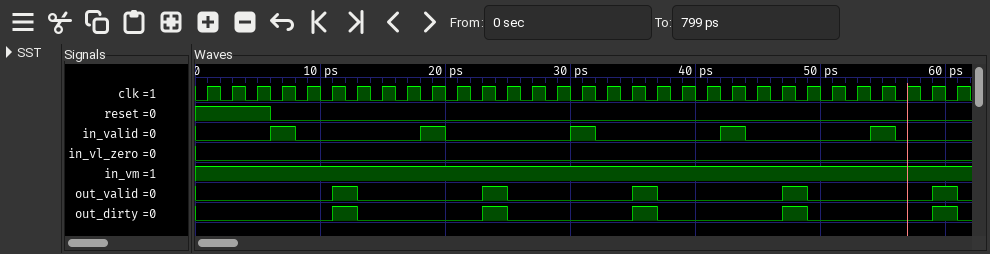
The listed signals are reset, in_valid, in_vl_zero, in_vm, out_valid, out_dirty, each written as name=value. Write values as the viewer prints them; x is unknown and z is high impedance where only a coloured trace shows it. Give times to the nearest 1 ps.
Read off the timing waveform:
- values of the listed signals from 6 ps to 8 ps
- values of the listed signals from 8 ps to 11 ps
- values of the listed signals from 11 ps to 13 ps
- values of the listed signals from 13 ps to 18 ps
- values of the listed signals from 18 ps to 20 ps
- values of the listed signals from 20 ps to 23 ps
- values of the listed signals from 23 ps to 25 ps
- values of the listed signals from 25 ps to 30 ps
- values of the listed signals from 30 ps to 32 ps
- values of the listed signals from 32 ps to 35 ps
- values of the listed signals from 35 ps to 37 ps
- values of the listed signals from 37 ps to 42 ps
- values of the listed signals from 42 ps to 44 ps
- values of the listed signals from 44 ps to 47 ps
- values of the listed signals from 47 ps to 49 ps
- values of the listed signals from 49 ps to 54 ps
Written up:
reset=0, in_valid=1, in_vl_zero=0, in_vm=1, out_valid=0, out_dirty=0
reset=0, in_valid=0, in_vl_zero=0, in_vm=1, out_valid=0, out_dirty=0
reset=0, in_valid=0, in_vl_zero=0, in_vm=1, out_valid=1, out_dirty=1
reset=0, in_valid=0, in_vl_zero=0, in_vm=1, out_valid=0, out_dirty=0
reset=0, in_valid=1, in_vl_zero=0, in_vm=1, out_valid=0, out_dirty=0
reset=0, in_valid=0, in_vl_zero=0, in_vm=1, out_valid=0, out_dirty=0
reset=0, in_valid=0, in_vl_zero=0, in_vm=1, out_valid=1, out_dirty=1
reset=0, in_valid=0, in_vl_zero=0, in_vm=1, out_valid=0, out_dirty=0
reset=0, in_valid=1, in_vl_zero=0, in_vm=1, out_valid=0, out_dirty=0
reset=0, in_valid=0, in_vl_zero=0, in_vm=1, out_valid=0, out_dirty=0
reset=0, in_valid=0, in_vl_zero=0, in_vm=1, out_valid=1, out_dirty=1
reset=0, in_valid=0, in_vl_zero=0, in_vm=1, out_valid=0, out_dirty=0
reset=0, in_valid=1, in_vl_zero=0, in_vm=1, out_valid=0, out_dirty=0
reset=0, in_valid=0, in_vl_zero=0, in_vm=1, out_valid=0, out_dirty=0
reset=0, in_valid=0, in_vl_zero=0, in_vm=1, out_valid=1, out_dirty=1
reset=0, in_valid=0, in_vl_zero=0, in_vm=1, out_valid=0, out_dirty=0
